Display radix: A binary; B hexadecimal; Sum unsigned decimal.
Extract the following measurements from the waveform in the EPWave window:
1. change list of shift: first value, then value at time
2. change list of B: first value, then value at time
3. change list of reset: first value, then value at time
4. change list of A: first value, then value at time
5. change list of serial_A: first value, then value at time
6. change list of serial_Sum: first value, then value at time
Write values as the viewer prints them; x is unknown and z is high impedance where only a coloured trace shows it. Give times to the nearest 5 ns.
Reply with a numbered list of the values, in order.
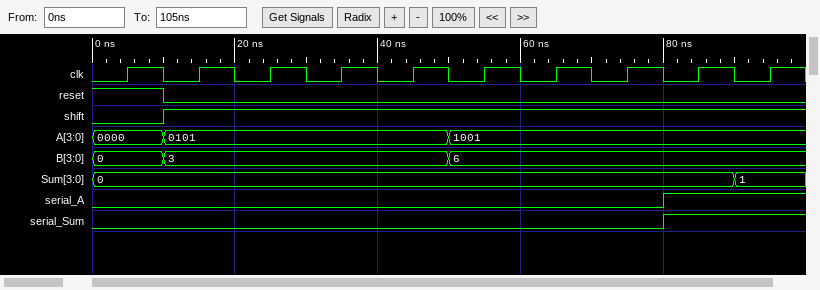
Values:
1. 0, 1 at 10 ns
2. 0, 3 at 10 ns, 6 at 50 ns
3. 1, 0 at 10 ns
4. 0000, 0101 at 10 ns, 1001 at 50 ns
5. 0, 1 at 80 ns
6. 0, 1 at 80 ns
